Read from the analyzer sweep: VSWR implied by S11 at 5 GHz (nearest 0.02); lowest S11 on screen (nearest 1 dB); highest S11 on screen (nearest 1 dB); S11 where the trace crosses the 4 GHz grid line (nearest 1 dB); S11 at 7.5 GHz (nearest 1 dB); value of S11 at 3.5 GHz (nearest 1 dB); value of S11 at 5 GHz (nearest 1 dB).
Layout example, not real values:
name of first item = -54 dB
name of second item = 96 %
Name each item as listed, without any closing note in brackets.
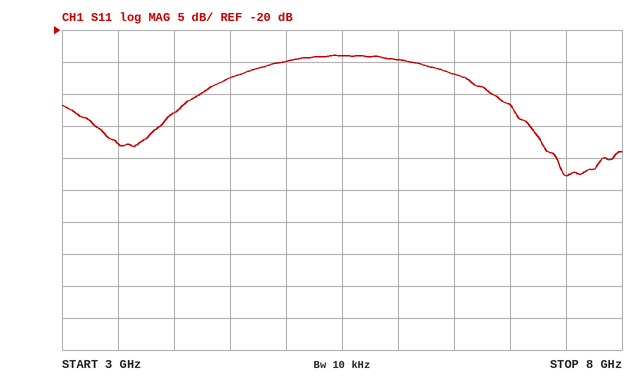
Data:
VSWR implied by S11 at 5 GHz = 1.12
lowest S11 on screen = -43 dB
highest S11 on screen = -24 dB
S11 where the trace crosses the 4 GHz grid line = -33 dB
S11 at 7.5 GHz = -43 dB
value of S11 at 3.5 GHz = -38 dB
value of S11 at 5 GHz = -25 dB
